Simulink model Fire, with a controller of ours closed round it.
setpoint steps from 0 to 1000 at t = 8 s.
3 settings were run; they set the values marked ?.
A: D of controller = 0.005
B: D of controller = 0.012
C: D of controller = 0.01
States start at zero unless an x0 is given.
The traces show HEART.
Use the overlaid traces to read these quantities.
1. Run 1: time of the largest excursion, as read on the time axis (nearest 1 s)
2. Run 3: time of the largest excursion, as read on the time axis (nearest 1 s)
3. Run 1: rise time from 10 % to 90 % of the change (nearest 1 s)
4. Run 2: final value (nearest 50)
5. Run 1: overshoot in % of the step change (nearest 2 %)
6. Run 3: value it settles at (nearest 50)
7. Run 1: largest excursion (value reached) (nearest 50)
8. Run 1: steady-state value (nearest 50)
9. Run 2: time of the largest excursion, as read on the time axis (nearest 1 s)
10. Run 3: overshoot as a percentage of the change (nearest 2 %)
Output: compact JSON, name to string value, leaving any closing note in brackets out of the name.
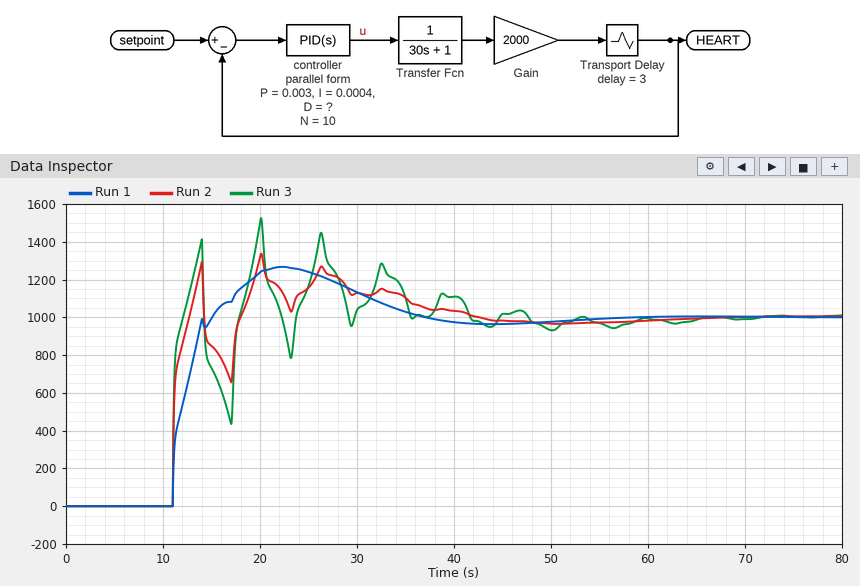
{"Run 1: time of the largest excursion, as read on the time axis": "22 s", "Run 3: time of the largest excursion, as read on the time axis": "20 s", "Run 1: rise time from 10 % to 90 % of the change": "3 s", "Run 2: final value": "1000", "Run 1: overshoot in % of the step change": "26 %", "Run 3: value it settles at": "1000", "Run 1: largest excursion (value reached)": "1250", "Run 1: steady-state value": "1000", "Run 2: time of the largest excursion, as read on the time axis": "20 s", "Run 3: overshoot as a percentage of the change": "52 %"}
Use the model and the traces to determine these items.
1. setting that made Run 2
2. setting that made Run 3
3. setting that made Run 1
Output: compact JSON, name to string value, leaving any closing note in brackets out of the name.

{"setting that made Run 2": "C", "setting that made Run 3": "B", "setting that made Run 1": "A"}
